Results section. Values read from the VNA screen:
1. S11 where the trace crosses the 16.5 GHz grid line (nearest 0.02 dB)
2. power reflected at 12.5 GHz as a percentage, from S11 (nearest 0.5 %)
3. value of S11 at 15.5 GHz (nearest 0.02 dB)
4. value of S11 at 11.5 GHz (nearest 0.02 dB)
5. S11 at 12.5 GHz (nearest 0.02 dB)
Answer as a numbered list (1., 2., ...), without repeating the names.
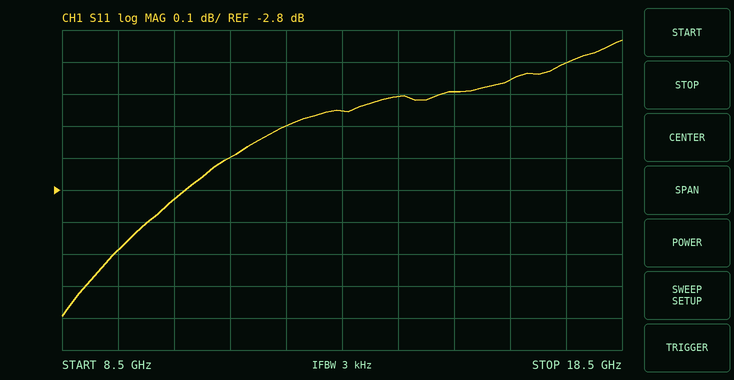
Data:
1. -2.46 dB
2. 55.0 %
3. -2.50 dB
4. -2.70 dB
5. -2.60 dB
